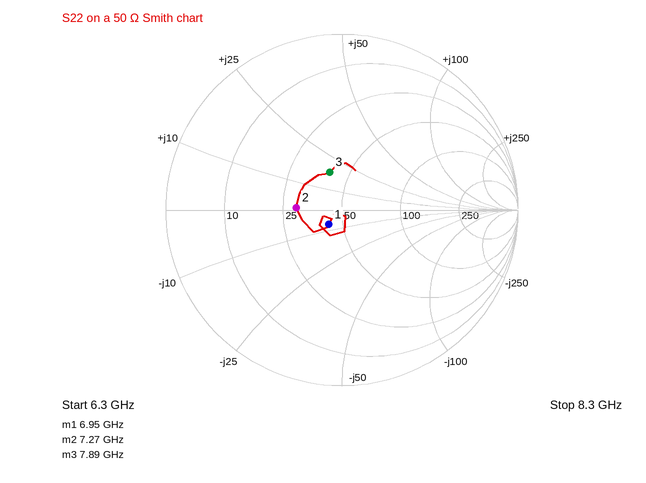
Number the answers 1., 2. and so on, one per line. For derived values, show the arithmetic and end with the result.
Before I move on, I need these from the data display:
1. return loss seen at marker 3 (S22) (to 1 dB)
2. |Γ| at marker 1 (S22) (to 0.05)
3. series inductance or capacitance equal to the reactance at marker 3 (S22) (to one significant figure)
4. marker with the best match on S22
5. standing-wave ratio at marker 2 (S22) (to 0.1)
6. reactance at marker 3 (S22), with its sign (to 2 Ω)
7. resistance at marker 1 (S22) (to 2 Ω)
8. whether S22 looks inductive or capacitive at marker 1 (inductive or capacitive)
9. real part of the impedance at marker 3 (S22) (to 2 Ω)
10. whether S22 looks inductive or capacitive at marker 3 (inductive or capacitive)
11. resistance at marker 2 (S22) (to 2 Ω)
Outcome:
1. 13 dB
2. 0.10
3. L = 18 Ω/(2π × 7.89 GHz) ≈ 363 pH, so 400 pH to one significant figure
4. marker 1
5. 1.7
6. +18 Ω
7. 42 Ω
8. capacitive
9. 40 Ω
10. inductive
11. 30 Ω
